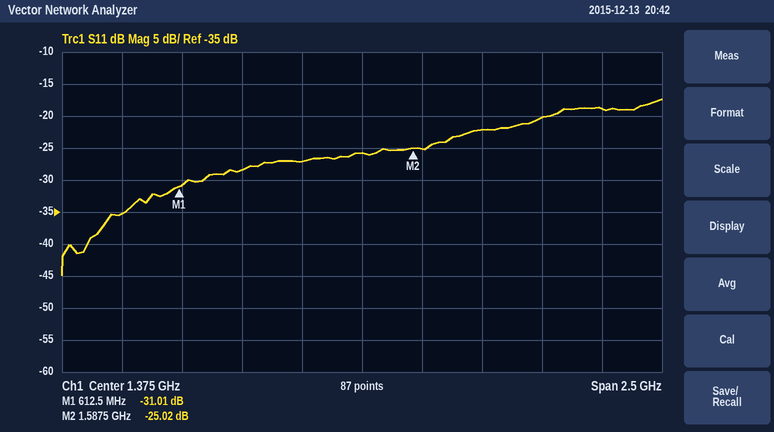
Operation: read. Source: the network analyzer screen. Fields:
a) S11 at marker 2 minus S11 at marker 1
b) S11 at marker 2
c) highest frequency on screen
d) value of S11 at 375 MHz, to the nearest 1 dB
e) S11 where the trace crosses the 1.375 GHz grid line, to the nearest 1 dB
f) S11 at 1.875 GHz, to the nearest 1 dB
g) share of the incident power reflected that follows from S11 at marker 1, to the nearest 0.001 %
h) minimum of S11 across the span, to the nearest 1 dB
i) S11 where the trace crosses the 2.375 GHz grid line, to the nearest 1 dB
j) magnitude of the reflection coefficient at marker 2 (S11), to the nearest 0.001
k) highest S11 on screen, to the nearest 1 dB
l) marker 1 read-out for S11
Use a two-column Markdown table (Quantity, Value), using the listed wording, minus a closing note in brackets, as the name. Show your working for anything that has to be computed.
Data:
| Quantity | Value |
|---|---|
| S11 at marker 2 minus S11 at marker 1 | -25.02 − (-31.01) = 5.99 dB |
| S11 at marker 2 | -25.02 dB |
| highest frequency on screen | 2.625 GHz |
| value of S11 at 375 MHz, to the nearest 1 dB | -35 dB |
| S11 where the trace crosses the 1.375 GHz grid line, to the nearest 1 dB | -26 dB |
| S11 at 1.875 GHz, to the nearest 1 dB | -22 dB |
| share of the incident power reflected that follows from S11 at marker 1, to the nearest 0.001 % | 10^(-31.01/10) ≈ 0.079 % |
| minimum of S11 across the span, to the nearest 1 dB | -45 dB |
| S11 where the trace crosses the 2.375 GHz grid line, to the nearest 1 dB | -19 dB |
| magnitude of the reflection coefficient at marker 2 (S11), to the nearest 0.001 | 10^(-25.02/20) ≈ 0.056 |
| highest S11 on screen, to the nearest 1 dB | -17 dB |
| marker 1 read-out for S11 | -31.01 dB |
